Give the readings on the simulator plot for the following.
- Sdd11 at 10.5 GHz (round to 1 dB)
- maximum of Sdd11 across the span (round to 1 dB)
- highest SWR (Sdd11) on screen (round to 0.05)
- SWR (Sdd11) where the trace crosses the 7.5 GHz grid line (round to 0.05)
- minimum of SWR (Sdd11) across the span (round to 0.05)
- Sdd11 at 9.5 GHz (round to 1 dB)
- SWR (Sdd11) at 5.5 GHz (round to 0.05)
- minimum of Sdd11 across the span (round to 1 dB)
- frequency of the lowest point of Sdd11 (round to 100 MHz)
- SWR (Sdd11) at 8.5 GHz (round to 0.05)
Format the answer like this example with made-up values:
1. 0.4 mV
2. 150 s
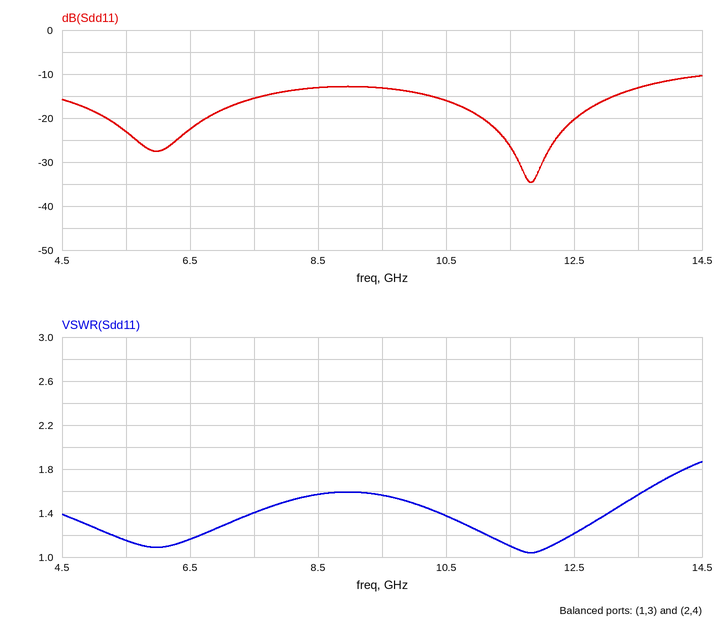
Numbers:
1. -16 dB
2. -10 dB
3. 1.85
4. 1.40
5. 1.05
6. -13 dB
7. 1.15
8. -35 dB
9. 11.8 GHz
10. 1.55
